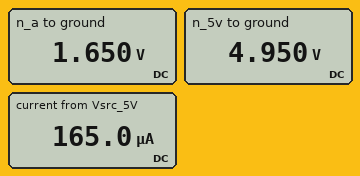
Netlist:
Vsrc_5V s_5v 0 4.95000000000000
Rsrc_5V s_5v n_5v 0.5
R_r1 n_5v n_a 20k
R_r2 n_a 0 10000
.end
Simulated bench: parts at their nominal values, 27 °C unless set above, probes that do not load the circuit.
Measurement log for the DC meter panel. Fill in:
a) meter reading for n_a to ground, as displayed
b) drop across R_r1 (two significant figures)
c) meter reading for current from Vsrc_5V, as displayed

1.650 V
3.3 V
165.0 µA
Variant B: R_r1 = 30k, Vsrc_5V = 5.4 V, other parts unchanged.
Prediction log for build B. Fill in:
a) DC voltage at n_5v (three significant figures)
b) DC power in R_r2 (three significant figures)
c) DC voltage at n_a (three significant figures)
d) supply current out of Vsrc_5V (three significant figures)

5.40 V
182 µW
1.35 V
135 µA
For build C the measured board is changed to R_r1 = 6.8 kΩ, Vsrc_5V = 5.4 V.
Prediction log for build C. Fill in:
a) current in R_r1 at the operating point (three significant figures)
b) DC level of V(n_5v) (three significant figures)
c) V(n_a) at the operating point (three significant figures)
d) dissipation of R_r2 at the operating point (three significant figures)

321 µA
5.40 V
3.21 V
1.03 mW
